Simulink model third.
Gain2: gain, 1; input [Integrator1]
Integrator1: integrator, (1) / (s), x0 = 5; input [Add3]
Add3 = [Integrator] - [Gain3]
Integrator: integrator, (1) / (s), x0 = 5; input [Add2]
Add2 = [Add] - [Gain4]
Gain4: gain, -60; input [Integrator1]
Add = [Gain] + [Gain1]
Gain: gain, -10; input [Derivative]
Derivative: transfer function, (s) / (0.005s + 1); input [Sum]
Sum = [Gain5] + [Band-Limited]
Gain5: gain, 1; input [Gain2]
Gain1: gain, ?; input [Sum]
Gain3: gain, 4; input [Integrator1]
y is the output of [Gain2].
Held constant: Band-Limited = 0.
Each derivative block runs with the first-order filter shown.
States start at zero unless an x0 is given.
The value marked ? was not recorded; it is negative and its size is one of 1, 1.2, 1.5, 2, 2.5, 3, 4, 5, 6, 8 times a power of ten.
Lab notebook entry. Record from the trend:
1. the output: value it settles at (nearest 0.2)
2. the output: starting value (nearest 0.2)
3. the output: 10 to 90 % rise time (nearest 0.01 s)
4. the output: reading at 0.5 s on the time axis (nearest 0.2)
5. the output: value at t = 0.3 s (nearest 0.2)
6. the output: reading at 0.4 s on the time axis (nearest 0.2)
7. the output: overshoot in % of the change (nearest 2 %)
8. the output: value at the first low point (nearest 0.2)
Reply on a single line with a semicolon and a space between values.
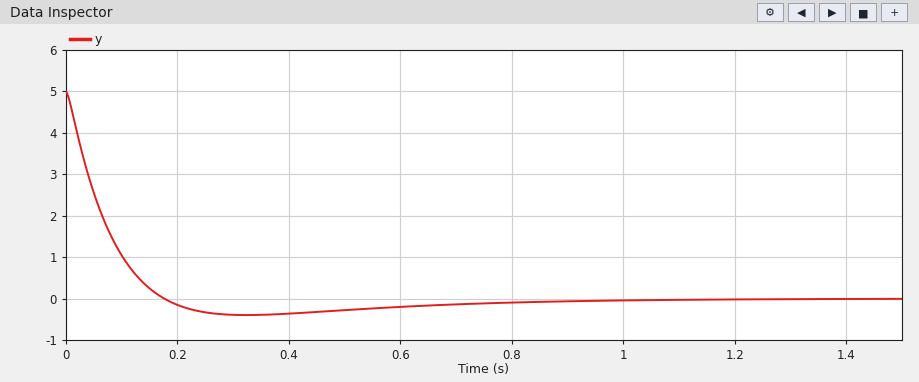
0.0; 5.0; 0.12 s; -0.2; -0.4; -0.4; 8 %; -0.4
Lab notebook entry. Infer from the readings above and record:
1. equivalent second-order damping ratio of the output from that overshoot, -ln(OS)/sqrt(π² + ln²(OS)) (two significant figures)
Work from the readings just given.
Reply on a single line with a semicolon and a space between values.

0.63
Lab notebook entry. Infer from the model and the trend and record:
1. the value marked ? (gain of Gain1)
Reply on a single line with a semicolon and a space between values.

-100
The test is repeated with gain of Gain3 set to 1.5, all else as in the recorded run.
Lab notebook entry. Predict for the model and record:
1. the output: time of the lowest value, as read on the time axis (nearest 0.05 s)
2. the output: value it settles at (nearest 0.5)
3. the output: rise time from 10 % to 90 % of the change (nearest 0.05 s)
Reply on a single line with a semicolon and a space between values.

0.35 s; 0.0; 0.15 s
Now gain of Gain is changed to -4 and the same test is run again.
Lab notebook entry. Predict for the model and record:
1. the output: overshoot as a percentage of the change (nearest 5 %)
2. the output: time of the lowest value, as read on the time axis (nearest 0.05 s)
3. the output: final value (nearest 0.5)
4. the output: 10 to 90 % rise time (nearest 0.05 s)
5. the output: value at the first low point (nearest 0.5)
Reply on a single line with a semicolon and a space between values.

20 %; 0.40 s; 0.0; 0.15 s; -1.0
